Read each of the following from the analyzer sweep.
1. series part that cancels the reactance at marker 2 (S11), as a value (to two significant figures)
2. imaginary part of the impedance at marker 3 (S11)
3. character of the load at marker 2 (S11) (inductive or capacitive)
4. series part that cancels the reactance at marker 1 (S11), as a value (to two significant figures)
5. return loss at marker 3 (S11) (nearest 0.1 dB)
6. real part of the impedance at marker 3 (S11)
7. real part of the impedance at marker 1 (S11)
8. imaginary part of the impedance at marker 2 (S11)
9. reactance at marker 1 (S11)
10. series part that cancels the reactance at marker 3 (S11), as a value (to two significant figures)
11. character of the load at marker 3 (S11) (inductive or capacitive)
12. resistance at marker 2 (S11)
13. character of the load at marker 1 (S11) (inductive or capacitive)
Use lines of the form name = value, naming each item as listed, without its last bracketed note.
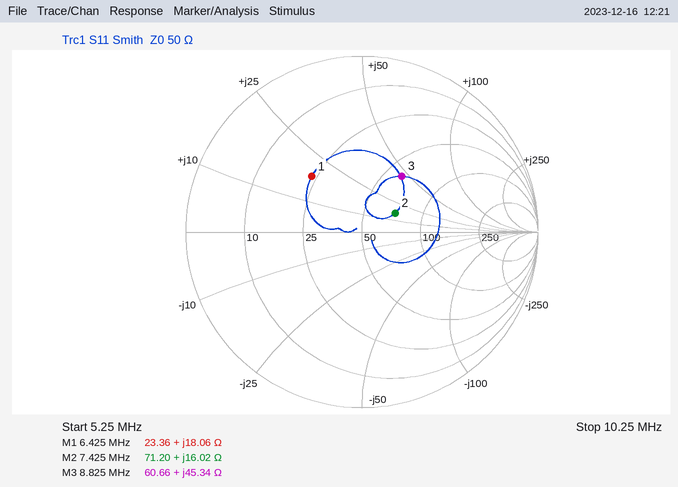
series part that cancels the reactance at marker 2 (S11), as a value = 1.3 nF
imaginary part of the impedance at marker 3 = +45.34 Ω
character of the load at marker 2 (S11) = inductive
series part that cancels the reactance at marker 1 (S11), as a value = 1.4 nF
return loss at marker 3 (S11) = 8.2 dB
real part of the impedance at marker 3 = 60.66 Ω
real part of the impedance at marker 1 = 23.36 Ω
imaginary part of the impedance at marker 2 = +16.02 Ω
reactance at marker 1 = +18.06 Ω
series part that cancels the reactance at marker 3 (S11), as a value = 400 pF
character of the load at marker 3 (S11) = inductive
resistance at marker 2 = 71.20 Ω
character of the load at marker 1 (S11) = inductive
